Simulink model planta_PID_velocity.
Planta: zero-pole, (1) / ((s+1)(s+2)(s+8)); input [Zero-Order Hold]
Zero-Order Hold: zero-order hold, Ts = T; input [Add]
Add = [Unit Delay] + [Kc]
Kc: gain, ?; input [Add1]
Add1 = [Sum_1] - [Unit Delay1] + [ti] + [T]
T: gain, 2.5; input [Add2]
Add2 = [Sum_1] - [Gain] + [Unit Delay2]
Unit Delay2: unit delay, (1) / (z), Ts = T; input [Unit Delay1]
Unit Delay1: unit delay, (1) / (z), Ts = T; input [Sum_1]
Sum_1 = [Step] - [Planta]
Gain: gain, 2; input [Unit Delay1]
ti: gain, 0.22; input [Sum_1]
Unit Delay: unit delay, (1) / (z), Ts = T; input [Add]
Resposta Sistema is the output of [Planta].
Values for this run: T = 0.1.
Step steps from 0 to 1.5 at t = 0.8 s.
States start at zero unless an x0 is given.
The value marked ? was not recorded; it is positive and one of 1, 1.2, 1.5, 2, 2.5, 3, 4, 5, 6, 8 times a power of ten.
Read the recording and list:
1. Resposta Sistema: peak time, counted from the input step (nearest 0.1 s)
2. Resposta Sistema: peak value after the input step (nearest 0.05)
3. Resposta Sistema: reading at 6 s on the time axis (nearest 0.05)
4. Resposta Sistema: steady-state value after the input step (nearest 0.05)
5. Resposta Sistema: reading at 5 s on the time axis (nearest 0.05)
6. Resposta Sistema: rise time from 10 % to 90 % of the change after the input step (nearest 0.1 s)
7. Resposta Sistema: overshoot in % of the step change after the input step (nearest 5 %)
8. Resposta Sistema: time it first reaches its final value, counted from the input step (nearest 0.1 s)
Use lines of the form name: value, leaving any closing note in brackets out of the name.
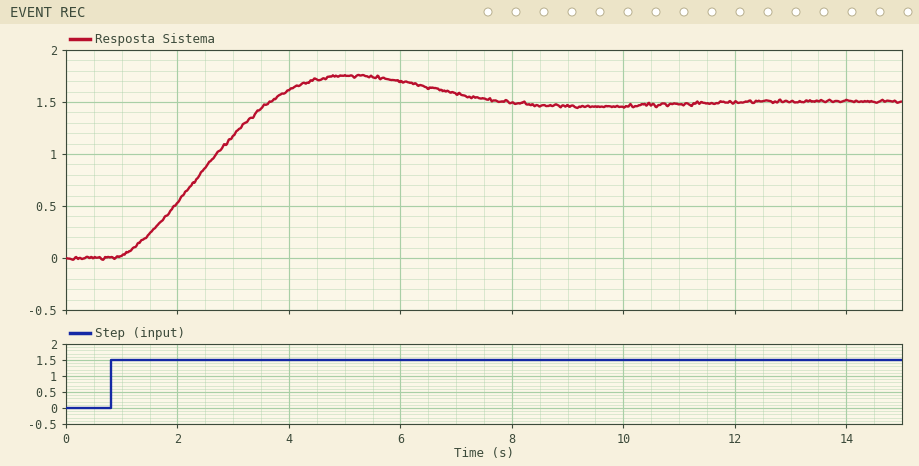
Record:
Resposta Sistema: peak time, counted from the input step: 4.3 s
Resposta Sistema: peak value after the input step: 1.75
Resposta Sistema: reading at 6 s on the time axis: 1.70
Resposta Sistema: steady-state value after the input step: 1.50
Resposta Sistema: reading at 5 s on the time axis: 1.75
Resposta Sistema: rise time from 10 % to 90 % of the change after the input step: 2.0 s
Resposta Sistema: overshoot in % of the step change after the input step: 15 %
Resposta Sistema: time it first reaches its final value, counted from the input step: 2.9 s
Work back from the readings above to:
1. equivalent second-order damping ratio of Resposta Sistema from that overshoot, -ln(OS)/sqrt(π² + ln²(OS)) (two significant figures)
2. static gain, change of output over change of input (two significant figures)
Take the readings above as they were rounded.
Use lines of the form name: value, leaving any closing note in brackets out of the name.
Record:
equivalent second-order damping ratio of Resposta Sistema from that overshoot, -ln(OS)/sqrt(π² + ln²(OS)): 0.52
static gain, change of output over change of input: 1.0
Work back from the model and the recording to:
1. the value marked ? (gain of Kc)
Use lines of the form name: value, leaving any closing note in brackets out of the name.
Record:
the value marked ?: 6
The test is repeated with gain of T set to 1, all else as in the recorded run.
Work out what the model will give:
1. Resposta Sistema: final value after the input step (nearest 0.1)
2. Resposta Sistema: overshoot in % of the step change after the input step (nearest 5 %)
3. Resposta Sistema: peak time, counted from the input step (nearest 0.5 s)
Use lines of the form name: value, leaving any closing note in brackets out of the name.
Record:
Resposta Sistema: final value after the input step: 1.5
Resposta Sistema: overshoot in % of the step change after the input step: 20 %
Resposta Sistema: peak time, counted from the input step: 4.0 s
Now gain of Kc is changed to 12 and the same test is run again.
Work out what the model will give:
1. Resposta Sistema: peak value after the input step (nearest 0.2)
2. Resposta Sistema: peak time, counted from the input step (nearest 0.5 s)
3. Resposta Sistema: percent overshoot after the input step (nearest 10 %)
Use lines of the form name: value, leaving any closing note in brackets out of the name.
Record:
Resposta Sistema: peak value after the input step: 2.0
Resposta Sistema: peak time, counted from the input step: 3.0 s
Resposta Sistema: percent overshoot after the input step: 30 %
